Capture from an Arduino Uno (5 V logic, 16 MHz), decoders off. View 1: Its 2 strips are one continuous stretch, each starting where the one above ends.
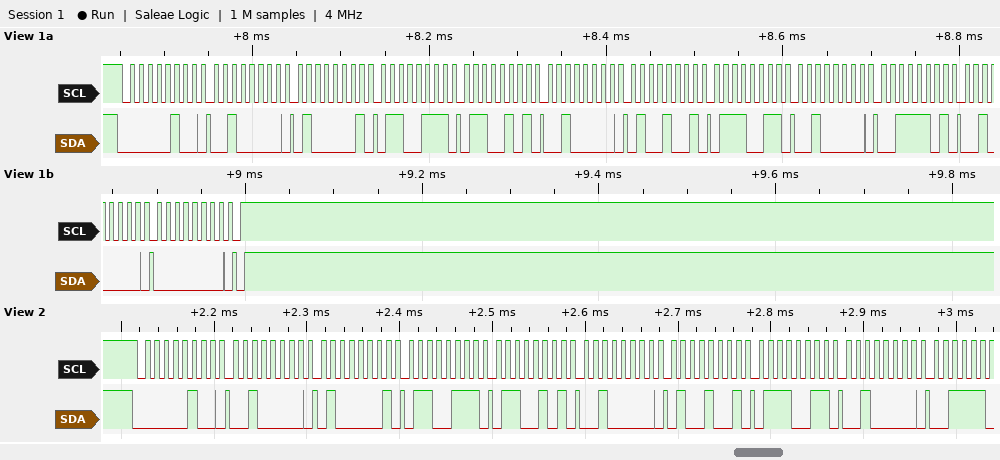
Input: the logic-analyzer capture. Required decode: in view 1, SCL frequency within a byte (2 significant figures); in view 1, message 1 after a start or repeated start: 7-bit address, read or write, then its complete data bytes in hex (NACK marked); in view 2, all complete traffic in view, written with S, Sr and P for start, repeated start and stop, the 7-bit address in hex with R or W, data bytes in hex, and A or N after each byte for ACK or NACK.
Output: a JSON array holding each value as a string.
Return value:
["100 kHz", "0x02 write: 20 41 67 65 20 49 73 20 3D 20 00", "S 02W A 20 A 41 A 67 A 65 A 20 A 49 A 73 A 20 A"]
